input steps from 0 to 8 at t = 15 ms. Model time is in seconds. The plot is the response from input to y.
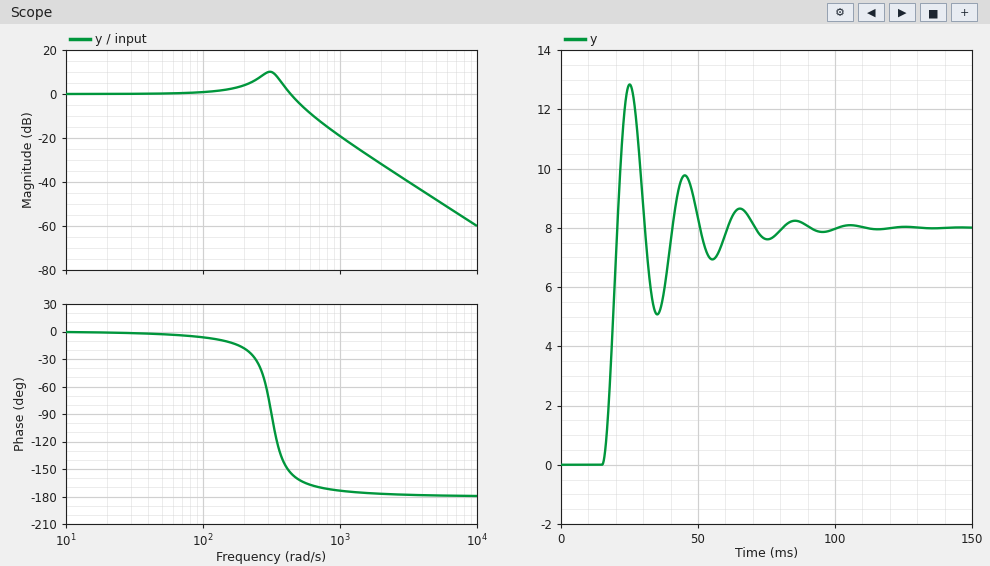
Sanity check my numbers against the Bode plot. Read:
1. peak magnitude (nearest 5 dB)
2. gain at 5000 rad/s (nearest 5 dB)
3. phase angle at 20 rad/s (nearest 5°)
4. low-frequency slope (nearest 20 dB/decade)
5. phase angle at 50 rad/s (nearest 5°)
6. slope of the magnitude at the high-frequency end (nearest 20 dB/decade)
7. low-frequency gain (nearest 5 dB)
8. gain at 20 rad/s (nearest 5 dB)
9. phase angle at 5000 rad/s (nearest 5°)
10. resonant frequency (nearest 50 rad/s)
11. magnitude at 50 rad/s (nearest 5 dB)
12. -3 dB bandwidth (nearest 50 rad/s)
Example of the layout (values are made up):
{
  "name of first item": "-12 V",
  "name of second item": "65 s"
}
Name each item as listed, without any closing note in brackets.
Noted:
{
  "peak magnitude": "10 dB",
  "gain at 5000 rad/s": "-50 dB",
  "phase angle at 20 rad/s": "0°",
  "low-frequency slope": "0 dB/decade",
  "phase angle at 50 rad/s": "-5°",
  "slope of the magnitude at the high-frequency end": "-40 dB/decade",
  "low-frequency gain": "0 dB",
  "gain at 20 rad/s": "0 dB",
  "phase angle at 5000 rad/s": "-180°",
  "resonant frequency": "300 rad/s",
  "magnitude at 50 rad/s": "0 dB",
  "-3 dB bandwidth": "500 rad/s"
}
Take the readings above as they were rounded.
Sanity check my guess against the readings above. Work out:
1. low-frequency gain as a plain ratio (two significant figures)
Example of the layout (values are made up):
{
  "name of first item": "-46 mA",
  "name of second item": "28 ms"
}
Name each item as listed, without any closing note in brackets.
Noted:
{
  "low-frequency gain as a plain ratio": "1.0"
}
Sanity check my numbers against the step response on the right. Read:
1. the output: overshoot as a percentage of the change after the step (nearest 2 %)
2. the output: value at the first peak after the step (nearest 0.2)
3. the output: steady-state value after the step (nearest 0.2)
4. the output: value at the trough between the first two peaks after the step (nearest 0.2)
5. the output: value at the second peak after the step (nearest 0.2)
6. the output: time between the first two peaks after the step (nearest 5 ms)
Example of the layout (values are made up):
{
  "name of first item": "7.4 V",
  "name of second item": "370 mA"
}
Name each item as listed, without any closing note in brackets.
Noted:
{
  "the output: overshoot as a percentage of the change after the step": "60 %",
  "the output: value at the first peak after the step": "12.8",
  "the output: steady-state value after the step": "8.0",
  "the output: value at the trough between the first two peaks after the step": "5.0",
  "the output: value at the second peak after the step": "9.8",
  "the output: time between the first two peaks after the step": "20 ms"
}
